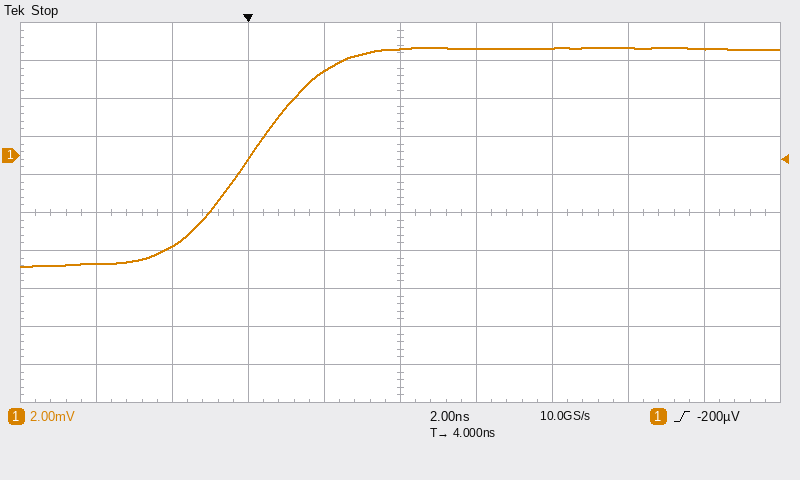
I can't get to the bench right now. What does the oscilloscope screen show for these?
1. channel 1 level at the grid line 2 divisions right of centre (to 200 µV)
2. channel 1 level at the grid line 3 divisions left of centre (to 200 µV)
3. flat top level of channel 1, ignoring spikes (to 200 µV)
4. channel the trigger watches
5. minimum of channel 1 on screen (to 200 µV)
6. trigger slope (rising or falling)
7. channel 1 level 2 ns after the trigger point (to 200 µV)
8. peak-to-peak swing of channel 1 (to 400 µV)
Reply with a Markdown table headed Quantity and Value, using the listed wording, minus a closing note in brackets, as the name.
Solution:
| Quantity | Value |
|---|---|
| channel 1 level at the grid line 2 divisions right of centre | 5.6 mV |
| channel 1 level at the grid line 3 divisions left of centre | -4.8 mV |
| flat top level of channel 1, ignoring spikes | 5.6 mV |
| channel the trigger watches | channel 1 |
| minimum of channel 1 on screen | -5.8 mV |
| trigger slope | rising |
| channel 1 level 2 ns after the trigger point | 4.4 mV |
| peak-to-peak swing of channel 1 | 11.6 mV |
